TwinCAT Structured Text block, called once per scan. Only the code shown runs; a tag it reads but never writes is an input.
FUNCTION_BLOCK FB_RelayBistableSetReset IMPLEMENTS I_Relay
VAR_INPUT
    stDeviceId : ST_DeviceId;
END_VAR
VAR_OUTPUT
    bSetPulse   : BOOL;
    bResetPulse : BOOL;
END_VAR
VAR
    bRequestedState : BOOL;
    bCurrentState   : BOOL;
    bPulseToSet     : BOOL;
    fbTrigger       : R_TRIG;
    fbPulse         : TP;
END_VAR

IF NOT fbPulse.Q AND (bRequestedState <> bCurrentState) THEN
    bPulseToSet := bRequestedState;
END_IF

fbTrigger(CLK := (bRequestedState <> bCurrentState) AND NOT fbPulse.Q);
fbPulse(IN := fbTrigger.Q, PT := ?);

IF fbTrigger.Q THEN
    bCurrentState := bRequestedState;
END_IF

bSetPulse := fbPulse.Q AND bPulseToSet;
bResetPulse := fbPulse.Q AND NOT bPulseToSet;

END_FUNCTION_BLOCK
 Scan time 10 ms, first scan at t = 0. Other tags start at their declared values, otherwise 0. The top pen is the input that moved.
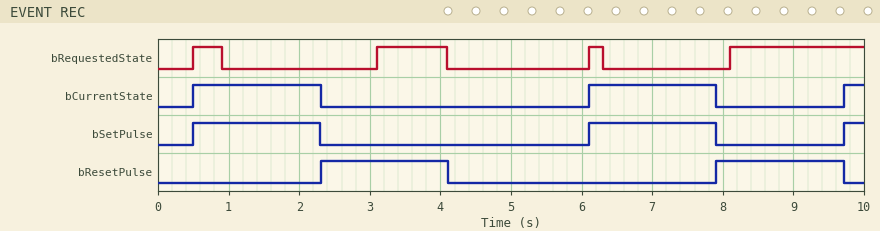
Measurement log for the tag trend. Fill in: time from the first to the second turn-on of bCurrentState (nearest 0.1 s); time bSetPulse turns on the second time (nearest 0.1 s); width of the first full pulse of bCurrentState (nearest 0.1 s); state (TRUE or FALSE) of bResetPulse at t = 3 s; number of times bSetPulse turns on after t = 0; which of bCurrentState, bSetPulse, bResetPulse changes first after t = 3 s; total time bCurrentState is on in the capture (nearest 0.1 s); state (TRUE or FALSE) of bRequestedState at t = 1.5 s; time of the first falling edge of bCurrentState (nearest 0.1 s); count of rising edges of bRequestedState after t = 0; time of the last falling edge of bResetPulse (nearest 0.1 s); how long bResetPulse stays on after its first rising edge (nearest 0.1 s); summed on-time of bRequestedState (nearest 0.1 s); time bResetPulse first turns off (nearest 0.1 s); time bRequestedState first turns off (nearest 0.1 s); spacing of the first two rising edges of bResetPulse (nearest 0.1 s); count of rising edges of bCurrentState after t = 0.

5.6 s
6.1 s
1.8 s
TRUE
3
bResetPulse
3.9 s
FALSE
2.3 s
4
9.7 s
1.8 s
3.5 s
4.1 s
0.9 s
5.6 s
3
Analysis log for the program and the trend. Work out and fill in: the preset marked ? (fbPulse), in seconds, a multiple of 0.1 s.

1.8 s
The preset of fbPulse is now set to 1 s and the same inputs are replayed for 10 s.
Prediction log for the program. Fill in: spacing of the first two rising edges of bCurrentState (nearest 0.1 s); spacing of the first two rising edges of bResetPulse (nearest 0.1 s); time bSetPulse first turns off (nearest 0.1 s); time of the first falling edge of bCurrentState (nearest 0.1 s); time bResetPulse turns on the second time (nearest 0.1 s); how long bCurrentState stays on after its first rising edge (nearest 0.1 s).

2.6 s
2.6 s
1.5 s
1.5 s
4.1 s
1.0 s
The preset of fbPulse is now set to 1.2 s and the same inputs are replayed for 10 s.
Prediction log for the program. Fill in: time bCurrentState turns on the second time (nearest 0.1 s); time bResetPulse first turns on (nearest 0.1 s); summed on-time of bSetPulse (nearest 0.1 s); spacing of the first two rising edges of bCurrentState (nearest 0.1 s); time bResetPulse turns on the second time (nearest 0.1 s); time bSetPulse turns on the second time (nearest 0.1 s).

3.1 s
1.7 s
4.8 s
2.6 s
4.3 s
3.1 s
